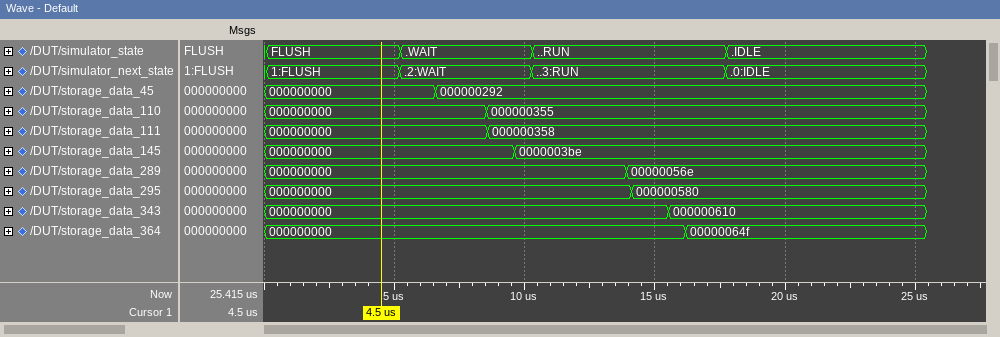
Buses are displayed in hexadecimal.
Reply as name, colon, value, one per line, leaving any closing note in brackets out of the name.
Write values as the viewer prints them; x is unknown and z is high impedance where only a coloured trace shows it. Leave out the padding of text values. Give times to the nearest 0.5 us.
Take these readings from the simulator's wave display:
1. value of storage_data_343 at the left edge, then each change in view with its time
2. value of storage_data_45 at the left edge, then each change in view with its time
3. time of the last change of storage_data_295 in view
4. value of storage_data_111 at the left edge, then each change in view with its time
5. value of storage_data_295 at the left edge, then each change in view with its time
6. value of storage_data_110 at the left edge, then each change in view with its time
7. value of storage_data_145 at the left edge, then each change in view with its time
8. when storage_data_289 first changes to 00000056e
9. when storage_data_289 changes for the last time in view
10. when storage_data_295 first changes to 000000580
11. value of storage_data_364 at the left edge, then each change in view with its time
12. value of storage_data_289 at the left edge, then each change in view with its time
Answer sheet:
value of storage_data_343 at the left edge, then each change in view with its time: 000000000, 000000610 at 15.5 us
value of storage_data_45 at the left edge, then each change in view with its time: 000000000, 000000292 at 6.5 us
time of the last change of storage_data_295 in view: 14 us
value of storage_data_111 at the left edge, then each change in view with its time: 000000000, 000000358 at 8.5 us
value of storage_data_295 at the left edge, then each change in view with its time: 000000000, 000000580 at 14 us
value of storage_data_110 at the left edge, then each change in view with its time: 000000000, 000000355 at 8.5 us
value of storage_data_145 at the left edge, then each change in view with its time: 000000000, 0000003be at 9.5 us
when storage_data_289 first changes to 00000056e: 14 us
when storage_data_289 changes for the last time in view: 14 us
when storage_data_295 first changes to 000000580: 14 us
value of storage_data_364 at the left edge, then each change in view with its time: 000000000, 00000064f at 16 us
value of storage_data_289 at the left edge, then each change in view with its time: 000000000, 00000056e at 14 us
